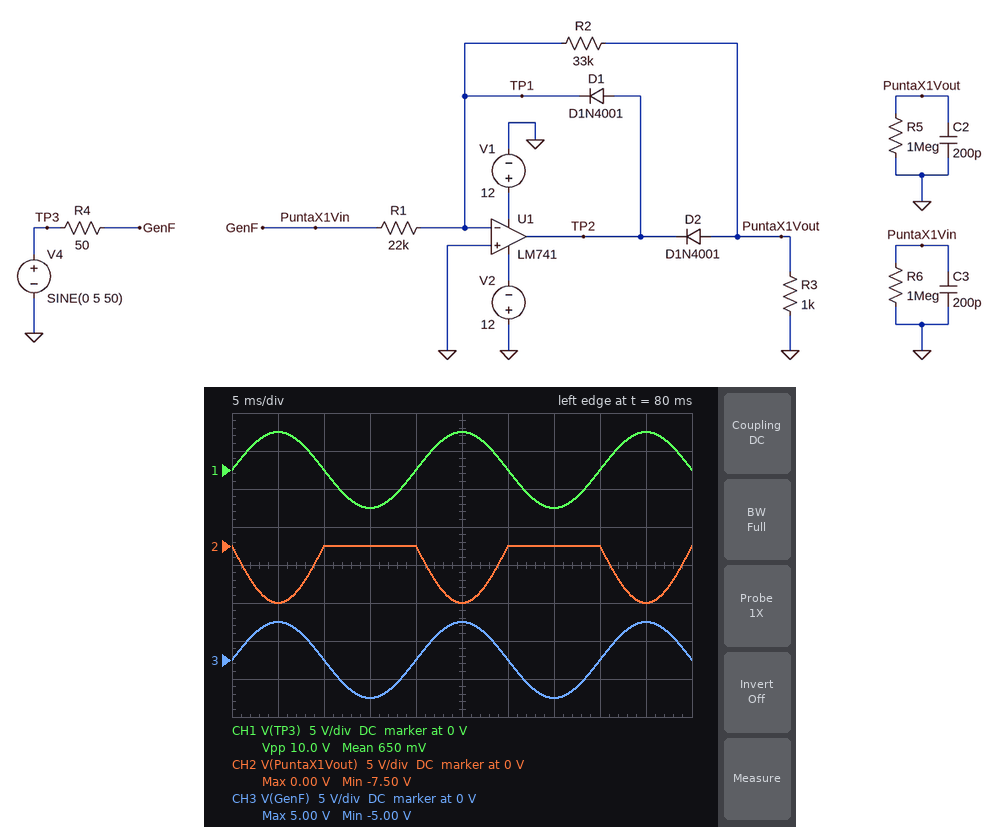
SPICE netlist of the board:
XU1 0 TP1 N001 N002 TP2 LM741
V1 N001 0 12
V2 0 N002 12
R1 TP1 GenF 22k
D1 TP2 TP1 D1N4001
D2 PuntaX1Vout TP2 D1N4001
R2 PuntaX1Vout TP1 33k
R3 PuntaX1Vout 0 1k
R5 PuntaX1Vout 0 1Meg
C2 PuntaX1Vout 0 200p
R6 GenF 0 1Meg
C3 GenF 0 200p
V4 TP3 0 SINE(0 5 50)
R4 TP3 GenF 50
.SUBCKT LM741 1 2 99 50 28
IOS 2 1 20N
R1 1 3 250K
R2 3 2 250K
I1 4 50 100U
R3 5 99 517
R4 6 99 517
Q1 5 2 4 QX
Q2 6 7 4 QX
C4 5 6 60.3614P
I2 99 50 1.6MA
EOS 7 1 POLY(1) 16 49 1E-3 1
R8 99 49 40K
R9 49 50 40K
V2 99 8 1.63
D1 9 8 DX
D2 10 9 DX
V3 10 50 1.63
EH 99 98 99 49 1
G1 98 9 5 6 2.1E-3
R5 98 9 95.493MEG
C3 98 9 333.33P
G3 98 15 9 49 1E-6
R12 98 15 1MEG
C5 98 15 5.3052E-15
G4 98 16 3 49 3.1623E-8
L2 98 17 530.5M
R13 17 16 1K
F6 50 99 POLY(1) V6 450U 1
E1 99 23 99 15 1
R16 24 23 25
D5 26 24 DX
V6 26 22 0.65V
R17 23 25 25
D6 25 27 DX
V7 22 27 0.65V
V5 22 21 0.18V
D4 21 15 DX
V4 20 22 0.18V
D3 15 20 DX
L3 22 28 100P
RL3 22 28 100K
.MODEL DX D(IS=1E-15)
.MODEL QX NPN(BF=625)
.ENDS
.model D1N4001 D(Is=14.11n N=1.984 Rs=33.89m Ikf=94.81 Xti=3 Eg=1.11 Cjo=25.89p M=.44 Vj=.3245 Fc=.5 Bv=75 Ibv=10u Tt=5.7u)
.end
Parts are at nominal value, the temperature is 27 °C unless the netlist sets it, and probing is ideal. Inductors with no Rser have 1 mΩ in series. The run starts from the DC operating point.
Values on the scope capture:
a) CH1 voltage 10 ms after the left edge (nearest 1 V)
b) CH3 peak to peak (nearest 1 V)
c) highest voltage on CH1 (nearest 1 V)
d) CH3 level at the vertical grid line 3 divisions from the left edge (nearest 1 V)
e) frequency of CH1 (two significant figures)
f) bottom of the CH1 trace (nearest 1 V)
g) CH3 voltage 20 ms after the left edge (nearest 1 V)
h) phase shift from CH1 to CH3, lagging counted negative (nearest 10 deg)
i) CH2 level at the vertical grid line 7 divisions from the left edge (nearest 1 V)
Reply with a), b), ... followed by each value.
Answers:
a) 0 V
b) 10 V
c) 5 V
d) -5 V
e) 50 Hz
f) -5 V
g) 0 V
h) 0 deg
i) 0 V
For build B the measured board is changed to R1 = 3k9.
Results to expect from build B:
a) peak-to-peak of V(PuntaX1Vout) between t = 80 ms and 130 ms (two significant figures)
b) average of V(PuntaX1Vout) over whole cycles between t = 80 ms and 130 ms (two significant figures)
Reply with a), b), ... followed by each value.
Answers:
a) 10 V
b) -4.6 V
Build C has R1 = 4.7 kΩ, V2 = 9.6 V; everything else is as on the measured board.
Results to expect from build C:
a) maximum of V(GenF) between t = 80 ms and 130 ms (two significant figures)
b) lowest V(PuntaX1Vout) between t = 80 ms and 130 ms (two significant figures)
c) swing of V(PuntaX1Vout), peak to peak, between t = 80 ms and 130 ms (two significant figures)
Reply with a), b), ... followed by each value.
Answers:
a) 5.0 V
b) -7.6 V
c) 7.7 V
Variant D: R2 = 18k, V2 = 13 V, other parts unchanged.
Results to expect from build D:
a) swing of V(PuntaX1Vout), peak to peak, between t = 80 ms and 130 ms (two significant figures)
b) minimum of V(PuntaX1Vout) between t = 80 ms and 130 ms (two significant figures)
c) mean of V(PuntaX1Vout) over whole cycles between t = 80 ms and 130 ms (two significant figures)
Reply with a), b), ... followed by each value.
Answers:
a) 4.1 V
b) -4.1 V
c) -1.3 V
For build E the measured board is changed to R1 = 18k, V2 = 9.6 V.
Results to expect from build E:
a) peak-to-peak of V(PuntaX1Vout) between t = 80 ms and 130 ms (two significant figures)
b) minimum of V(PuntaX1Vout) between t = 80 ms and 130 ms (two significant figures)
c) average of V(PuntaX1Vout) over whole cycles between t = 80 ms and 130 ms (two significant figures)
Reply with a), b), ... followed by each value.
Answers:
a) 7.6 V
b) -7.6 V
c) -2.7 V
